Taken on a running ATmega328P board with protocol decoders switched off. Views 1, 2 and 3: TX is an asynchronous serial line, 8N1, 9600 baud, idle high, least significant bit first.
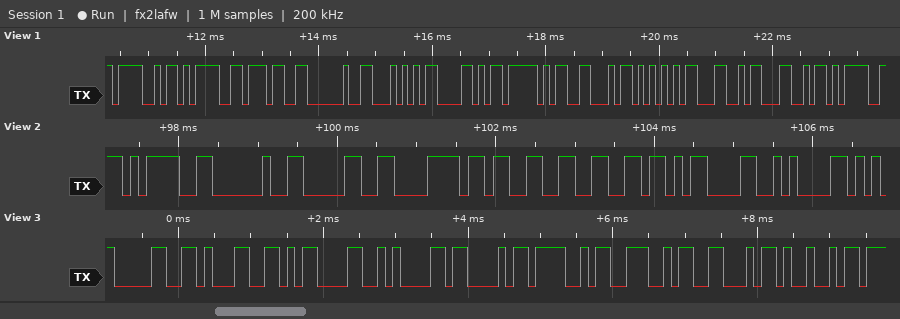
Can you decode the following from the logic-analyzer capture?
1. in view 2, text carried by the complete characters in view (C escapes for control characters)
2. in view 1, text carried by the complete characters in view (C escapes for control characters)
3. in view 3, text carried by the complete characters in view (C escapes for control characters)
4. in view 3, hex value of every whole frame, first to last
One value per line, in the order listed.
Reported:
"= 0x3f\r\n"
"O=7 TX_FULL="
"01\r\nCONFI"
30 31 0D 0A 43 4F 4E 46 49
